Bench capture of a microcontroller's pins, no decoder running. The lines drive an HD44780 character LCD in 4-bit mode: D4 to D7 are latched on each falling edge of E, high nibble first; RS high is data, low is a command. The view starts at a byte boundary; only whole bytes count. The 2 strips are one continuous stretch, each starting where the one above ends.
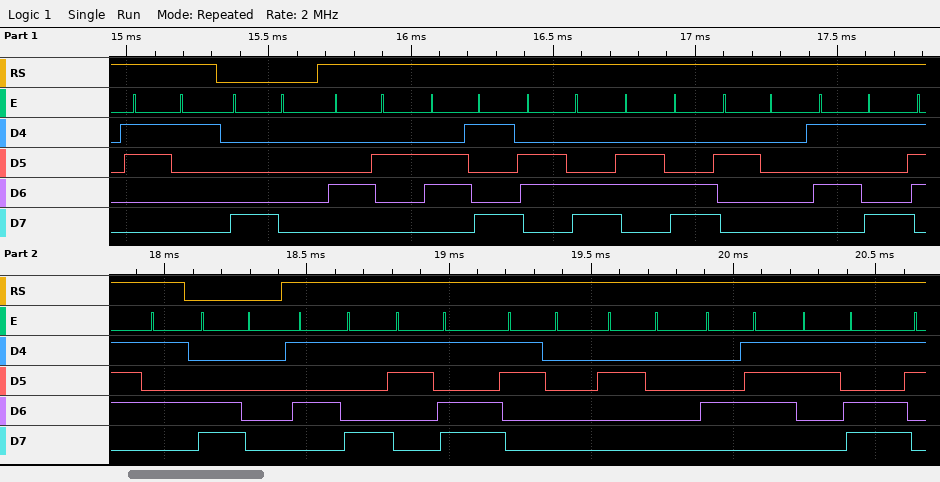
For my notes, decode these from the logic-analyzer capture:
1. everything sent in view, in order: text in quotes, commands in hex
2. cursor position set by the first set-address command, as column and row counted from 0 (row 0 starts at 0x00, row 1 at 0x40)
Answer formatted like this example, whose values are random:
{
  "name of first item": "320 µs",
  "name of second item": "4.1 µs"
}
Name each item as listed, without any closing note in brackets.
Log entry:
{
  "everything sent in view, in order: text in quotes, commands in hex": "\"1\" 0x80 \"Bill Yu\" 0xC0 \"Y=0 G=\"",
  "cursor position set by the first set-address command, as column and row counted from 0": "column 0, row 0"
}
